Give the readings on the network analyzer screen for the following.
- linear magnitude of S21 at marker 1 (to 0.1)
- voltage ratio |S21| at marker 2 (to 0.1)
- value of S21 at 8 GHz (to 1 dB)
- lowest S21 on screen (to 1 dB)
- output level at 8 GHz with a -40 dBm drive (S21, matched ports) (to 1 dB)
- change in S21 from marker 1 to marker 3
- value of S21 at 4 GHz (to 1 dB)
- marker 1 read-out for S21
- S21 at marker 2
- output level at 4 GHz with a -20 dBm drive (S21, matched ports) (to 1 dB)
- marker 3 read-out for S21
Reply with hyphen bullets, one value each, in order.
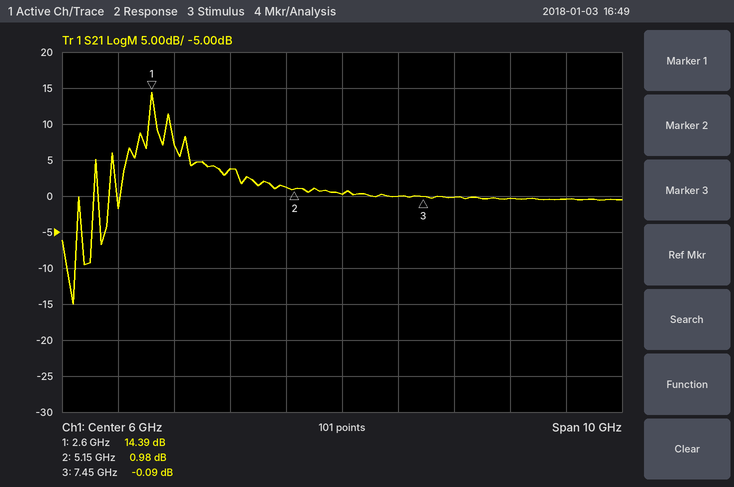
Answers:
- 5.2
- 1.1
- 0 dB
- -15 dB
- -40 dBm
- -14.48 dB
- 4 dB
- 14.39 dB
- 0.98 dB
- -16 dBm
- -0.09 dB
